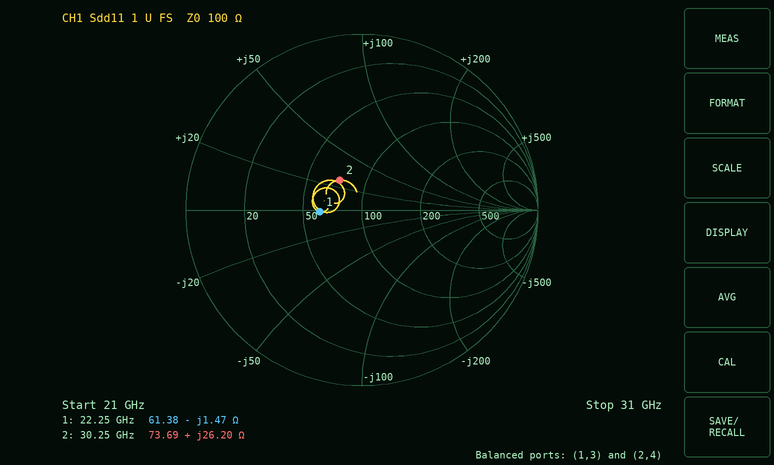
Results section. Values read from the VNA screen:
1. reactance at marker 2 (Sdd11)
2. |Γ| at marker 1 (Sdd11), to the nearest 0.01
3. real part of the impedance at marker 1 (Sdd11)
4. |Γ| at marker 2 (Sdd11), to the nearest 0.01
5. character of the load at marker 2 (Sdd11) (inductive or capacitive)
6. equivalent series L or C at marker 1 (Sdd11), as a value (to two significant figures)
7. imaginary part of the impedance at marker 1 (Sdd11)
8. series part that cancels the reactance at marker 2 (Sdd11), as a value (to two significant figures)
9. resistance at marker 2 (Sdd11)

+26.20 Ω
0.24
61.38 Ω
0.21
inductive
4.9 pF
-1.47 Ω
200 fF
73.69 Ω
